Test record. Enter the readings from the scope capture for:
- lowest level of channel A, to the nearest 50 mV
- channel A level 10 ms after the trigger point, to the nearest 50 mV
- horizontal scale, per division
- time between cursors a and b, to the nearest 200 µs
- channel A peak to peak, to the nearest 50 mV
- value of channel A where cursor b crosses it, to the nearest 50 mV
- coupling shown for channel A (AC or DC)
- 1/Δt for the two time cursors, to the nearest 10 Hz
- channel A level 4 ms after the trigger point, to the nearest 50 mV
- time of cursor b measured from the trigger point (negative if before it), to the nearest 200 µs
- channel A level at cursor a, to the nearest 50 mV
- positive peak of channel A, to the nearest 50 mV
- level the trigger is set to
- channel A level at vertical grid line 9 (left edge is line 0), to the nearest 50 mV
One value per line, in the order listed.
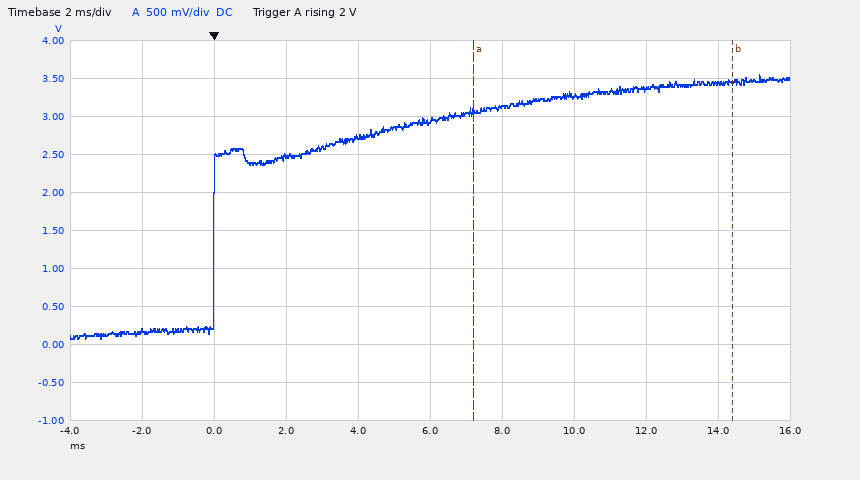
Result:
100 mV
3.25 V
2 ms
7.2 ms
3.45 V
3.45 V
DC
140 Hz
2.75 V
+14.4 ms
3.05 V
3.55 V
2 V
3.45 V
